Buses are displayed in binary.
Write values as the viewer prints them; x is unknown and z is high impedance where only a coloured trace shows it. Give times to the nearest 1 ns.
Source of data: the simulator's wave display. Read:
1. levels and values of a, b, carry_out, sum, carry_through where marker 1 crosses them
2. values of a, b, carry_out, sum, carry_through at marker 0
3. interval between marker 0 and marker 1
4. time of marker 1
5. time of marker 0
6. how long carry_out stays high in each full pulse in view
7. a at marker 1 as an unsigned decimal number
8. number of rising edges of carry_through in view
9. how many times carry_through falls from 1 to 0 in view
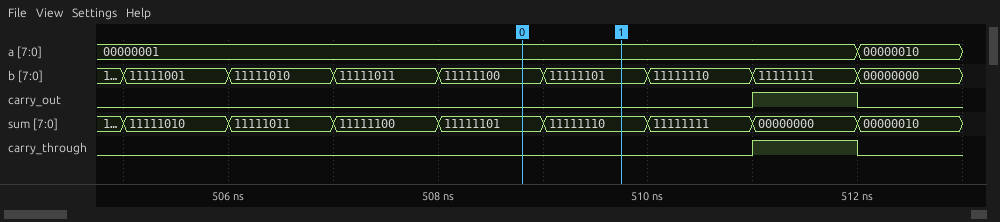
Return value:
a=00000001, b=11111101, carry_out=0, sum=11111110, carry_through=0
a=00000001, b=11111100, carry_out=0, sum=11111101, carry_through=0
1 ns
510 ns
509 ns
1 ns
1
1
1
